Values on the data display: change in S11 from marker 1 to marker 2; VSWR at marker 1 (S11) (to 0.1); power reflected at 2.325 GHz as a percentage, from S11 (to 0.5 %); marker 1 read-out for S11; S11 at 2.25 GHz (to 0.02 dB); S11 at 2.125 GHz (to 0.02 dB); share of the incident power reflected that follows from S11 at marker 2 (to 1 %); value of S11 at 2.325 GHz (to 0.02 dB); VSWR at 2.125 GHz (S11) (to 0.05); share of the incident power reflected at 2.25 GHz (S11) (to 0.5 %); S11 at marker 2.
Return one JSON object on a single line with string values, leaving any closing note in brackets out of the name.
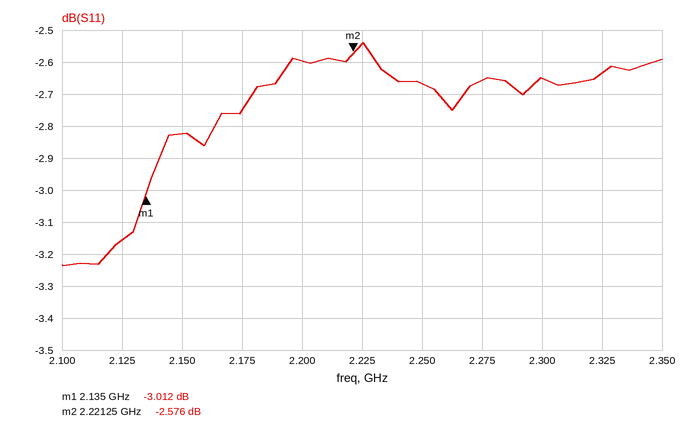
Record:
{"change in S11 from marker 1 to marker 2": "0.436 dB", "VSWR at marker 1 (S11)": "5.8", "power reflected at 2.325 GHz as a percentage, from S11": "54.5 %", "marker 1 read-out for S11": "-3.012 dB", "S11 at 2.25 GHz": "-2.66 dB", "S11 at 2.125 GHz": "-3.16 dB", "share of the incident power reflected that follows from S11 at marker 2": "55 %", "value of S11 at 2.325 GHz": "-2.64 dB", "VSWR at 2.125 GHz (S11)": "5.55", "share of the incident power reflected at 2.25 GHz (S11)": "54.0 %", "S11 at marker 2": "-2.576 dB"}
